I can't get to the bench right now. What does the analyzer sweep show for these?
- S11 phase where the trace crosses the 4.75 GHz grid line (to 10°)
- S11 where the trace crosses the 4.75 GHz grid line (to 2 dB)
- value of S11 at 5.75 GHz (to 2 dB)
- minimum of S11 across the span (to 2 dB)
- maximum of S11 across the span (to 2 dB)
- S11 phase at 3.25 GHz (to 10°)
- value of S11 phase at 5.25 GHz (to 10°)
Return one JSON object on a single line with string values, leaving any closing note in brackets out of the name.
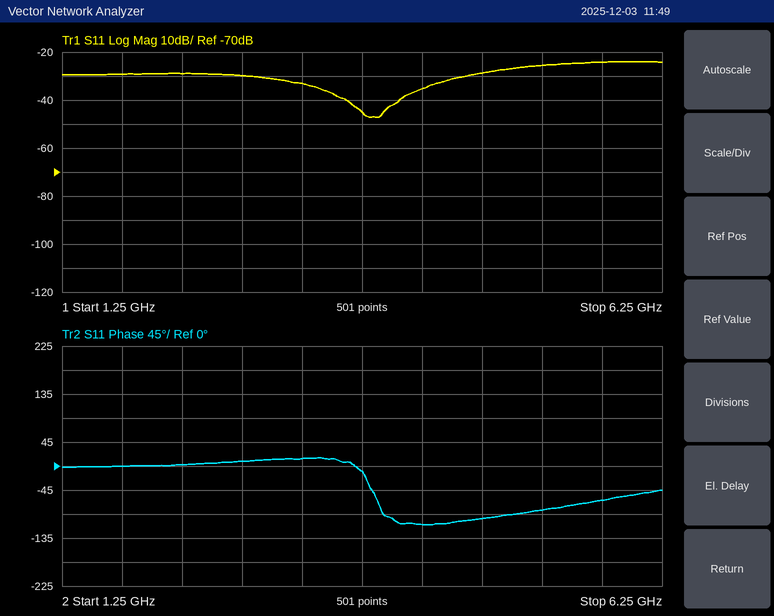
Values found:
{"S11 phase where the trace crosses the 4.75 GHz grid line": "-100°", "S11 where the trace crosses the 4.75 GHz grid line": "-28 dB", "value of S11 at 5.75 GHz": "-24 dB", "minimum of S11 across the span": "-48 dB", "maximum of S11 across the span": "-24 dB", "S11 phase at 3.25 GHz": "10°", "value of S11 phase at 5.25 GHz": "-80°"}
